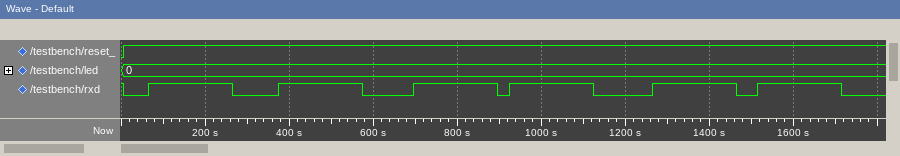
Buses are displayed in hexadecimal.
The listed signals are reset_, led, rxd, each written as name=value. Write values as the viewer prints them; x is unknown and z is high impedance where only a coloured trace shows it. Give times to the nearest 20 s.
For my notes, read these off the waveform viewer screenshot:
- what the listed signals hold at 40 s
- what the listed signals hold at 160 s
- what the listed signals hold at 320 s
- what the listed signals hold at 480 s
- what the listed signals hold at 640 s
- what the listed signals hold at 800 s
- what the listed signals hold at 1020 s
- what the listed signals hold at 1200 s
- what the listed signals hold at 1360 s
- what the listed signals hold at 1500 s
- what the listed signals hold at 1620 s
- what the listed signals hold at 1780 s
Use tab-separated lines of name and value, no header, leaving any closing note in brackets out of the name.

what the listed signals hold at 40 s	reset_=1, led=0, rxd=0
what the listed signals hold at 160 s	reset_=1, led=0, rxd=1
what the listed signals hold at 320 s	reset_=1, led=0, rxd=0
what the listed signals hold at 480 s	reset_=1, led=0, rxd=1
what the listed signals hold at 640 s	reset_=1, led=0, rxd=0
what the listed signals hold at 800 s	reset_=1, led=0, rxd=1
what the listed signals hold at 1020 s	reset_=1, led=0, rxd=1
what the listed signals hold at 1200 s	reset_=1, led=0, rxd=0
what the listed signals hold at 1360 s	reset_=1, led=0, rxd=1
what the listed signals hold at 1500 s	reset_=1, led=0, rxd=0
what the listed signals hold at 1620 s	reset_=1, led=0, rxd=1
what the listed signals hold at 1780 s	reset_=1, led=0, rxd=0
